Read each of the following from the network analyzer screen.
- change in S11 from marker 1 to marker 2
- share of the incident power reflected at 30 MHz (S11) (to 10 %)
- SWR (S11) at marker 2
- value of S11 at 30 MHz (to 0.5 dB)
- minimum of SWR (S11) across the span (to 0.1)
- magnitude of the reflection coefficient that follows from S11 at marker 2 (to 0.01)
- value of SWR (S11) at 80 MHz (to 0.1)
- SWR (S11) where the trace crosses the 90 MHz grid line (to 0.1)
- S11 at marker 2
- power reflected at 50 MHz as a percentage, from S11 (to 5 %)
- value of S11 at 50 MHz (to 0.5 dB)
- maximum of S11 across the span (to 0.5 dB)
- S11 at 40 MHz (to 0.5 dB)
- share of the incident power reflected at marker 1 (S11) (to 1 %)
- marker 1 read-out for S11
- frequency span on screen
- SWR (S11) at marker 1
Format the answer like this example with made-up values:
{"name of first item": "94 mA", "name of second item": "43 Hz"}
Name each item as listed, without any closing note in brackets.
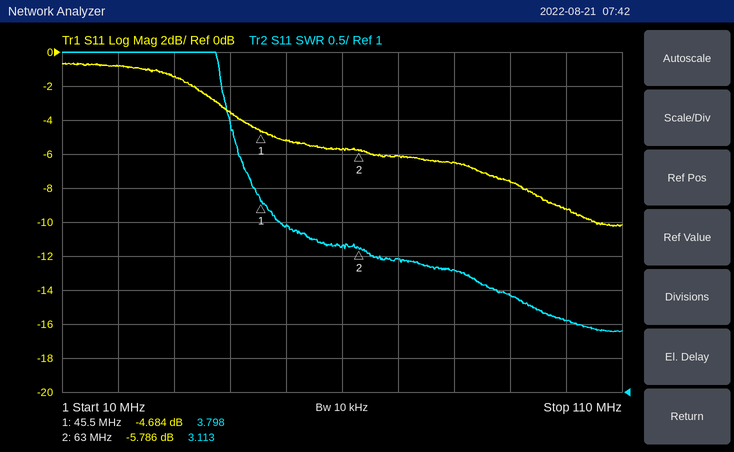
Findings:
{"change in S11 from marker 1 to marker 2": "-1.102 dB", "share of the incident power reflected at 30 MHz (S11)": "70 %", "SWR (S11) at marker 2": "3.113", "value of S11 at 30 MHz": "-1.5 dB", "minimum of SWR (S11) across the span": "1.9", "magnitude of the reflection coefficient that follows from S11 at marker 2": "0.51", "value of SWR (S11) at 80 MHz": "2.8", "SWR (S11) where the trace crosses the 90 MHz grid line": "2.4", "S11 at marker 2": "-5.786 dB", "power reflected at 50 MHz as a percentage, from S11": "30 %", "value of S11 at 50 MHz": "-5.0 dB", "maximum of S11 across the span": "-0.5 dB", "S11 at 40 MHz": "-3.5 dB", "share of the incident power reflected at marker 1 (S11)": "34 %", "marker 1 read-out for S11": "-4.684 dB", "frequency span on screen": "100 MHz", "SWR (S11) at marker 1": "3.798"}
